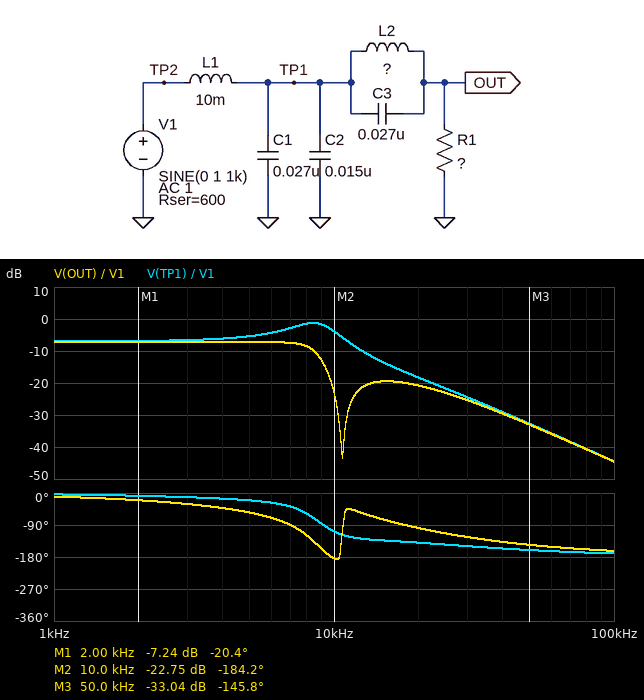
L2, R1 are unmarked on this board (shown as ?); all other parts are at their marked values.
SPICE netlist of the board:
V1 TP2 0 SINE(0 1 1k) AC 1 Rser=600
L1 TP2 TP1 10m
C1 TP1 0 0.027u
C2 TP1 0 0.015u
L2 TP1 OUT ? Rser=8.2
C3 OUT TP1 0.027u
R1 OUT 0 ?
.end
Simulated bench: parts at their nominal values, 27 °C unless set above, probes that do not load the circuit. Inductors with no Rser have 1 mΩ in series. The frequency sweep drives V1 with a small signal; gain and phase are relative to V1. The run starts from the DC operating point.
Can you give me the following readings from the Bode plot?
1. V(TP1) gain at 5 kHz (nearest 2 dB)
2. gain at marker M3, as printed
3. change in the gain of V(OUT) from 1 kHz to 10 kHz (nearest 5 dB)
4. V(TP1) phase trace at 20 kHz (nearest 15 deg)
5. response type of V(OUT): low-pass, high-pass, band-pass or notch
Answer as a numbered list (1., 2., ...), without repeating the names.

1. -6 dB
2. -33.04 dB
3. -15 dB
4. -135 deg
5. low-pass
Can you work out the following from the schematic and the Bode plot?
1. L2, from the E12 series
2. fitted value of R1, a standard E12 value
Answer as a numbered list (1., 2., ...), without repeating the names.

1. 8.2 mH
2. 470 Ω
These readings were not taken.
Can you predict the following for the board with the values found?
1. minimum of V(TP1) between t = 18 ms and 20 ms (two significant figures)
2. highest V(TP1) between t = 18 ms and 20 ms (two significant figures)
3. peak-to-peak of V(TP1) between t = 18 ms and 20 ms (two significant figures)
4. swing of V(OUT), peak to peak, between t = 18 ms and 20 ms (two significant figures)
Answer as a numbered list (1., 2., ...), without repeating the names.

1. -450 mV
2. 450 mV
3. 890 mV
4. 870 mV
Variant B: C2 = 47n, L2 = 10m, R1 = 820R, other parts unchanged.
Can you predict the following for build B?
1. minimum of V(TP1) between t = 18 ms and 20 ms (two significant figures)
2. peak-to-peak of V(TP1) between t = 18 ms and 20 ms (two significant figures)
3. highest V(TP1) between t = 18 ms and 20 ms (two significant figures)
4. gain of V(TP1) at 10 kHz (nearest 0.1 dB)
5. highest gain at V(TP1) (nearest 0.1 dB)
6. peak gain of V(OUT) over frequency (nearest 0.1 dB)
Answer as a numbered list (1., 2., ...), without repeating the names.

1. -580 mV
2. 1.2 V
3. 580 mV
4. -10.8 dB
5. -4.7 dB
6. -4.8 dB
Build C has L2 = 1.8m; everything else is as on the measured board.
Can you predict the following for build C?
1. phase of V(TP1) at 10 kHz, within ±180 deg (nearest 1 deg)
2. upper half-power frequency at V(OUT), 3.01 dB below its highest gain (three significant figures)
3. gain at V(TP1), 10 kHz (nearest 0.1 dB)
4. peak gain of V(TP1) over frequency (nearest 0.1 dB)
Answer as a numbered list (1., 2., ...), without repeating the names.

1. -71 deg
2. 12.4 kHz
3. -8.3 dB
4. -7.1 dB
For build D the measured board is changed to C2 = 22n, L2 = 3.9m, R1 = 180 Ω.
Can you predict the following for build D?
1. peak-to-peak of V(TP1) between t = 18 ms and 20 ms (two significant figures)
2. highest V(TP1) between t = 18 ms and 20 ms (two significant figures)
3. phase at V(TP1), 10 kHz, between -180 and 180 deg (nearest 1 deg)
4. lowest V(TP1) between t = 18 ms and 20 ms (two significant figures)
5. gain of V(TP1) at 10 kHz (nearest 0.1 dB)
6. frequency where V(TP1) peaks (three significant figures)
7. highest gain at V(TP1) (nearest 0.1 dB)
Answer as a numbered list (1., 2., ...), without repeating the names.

1. 480 mV
2. 240 mV
3. -57 deg
4. -240 mV
5. -3.7 dB
6. 10.6 kHz
7. -3.4 dB
